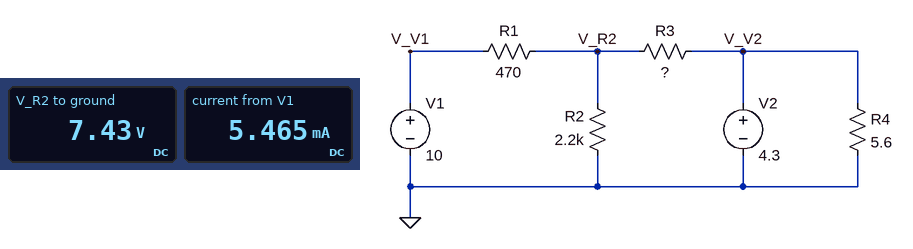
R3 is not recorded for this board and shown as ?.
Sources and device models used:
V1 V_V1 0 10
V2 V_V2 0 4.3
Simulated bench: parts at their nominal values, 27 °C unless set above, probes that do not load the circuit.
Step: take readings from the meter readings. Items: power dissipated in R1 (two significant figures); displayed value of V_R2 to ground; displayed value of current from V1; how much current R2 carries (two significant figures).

14 mW
7.43 V
5.465 mA
3.4 mA
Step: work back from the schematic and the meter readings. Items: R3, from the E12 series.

1.5 kΩ
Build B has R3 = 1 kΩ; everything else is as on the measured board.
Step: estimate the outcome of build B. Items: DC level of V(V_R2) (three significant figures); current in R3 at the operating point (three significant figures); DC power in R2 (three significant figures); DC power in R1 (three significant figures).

7.14 V
2.84 mA
23.2 mW
17.4 mW
